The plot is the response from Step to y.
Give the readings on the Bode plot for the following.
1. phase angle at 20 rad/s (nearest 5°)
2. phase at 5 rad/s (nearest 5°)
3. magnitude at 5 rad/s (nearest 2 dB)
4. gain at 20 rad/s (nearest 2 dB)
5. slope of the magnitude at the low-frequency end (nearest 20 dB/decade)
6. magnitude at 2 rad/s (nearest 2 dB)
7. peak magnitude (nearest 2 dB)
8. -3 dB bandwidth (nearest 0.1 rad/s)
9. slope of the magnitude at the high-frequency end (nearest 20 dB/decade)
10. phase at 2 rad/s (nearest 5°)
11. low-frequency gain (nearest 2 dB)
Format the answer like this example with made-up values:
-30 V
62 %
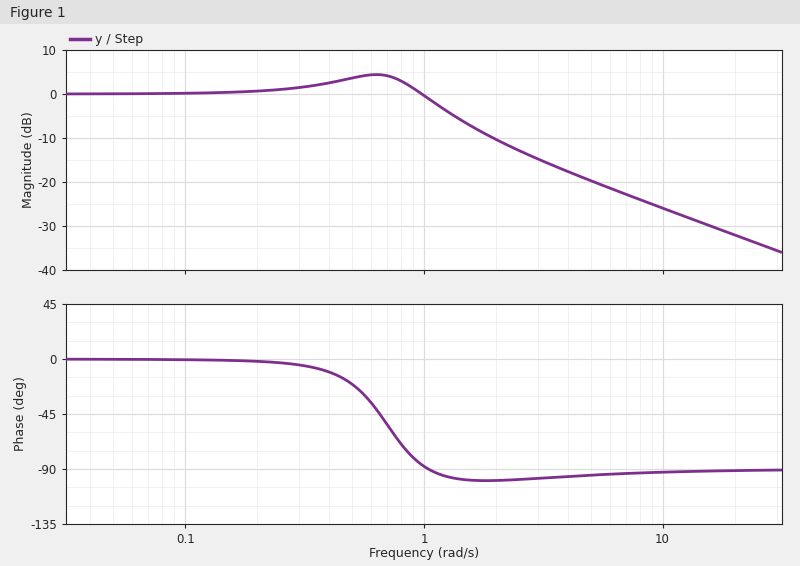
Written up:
-90°
-95°
-20 dB
-32 dB
0 dB/decade
-10 dB
4 dB
1.2 rad/s
-20 dB/decade
-100°
0 dB
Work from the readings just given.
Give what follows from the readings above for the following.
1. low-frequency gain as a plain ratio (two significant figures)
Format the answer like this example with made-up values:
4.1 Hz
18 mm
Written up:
1.0
